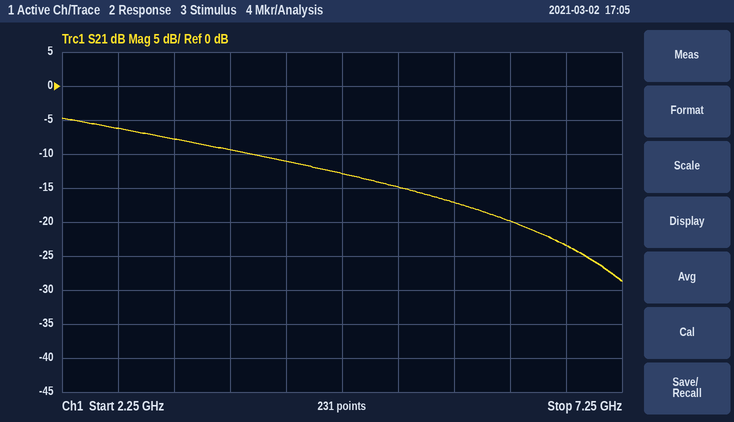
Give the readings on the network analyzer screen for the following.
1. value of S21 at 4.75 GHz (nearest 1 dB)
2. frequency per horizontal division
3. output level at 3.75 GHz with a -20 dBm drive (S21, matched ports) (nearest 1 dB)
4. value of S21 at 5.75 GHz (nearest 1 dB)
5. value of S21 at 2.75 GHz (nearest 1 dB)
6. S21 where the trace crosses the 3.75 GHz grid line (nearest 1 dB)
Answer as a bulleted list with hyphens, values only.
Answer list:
- -13 dB
- 500 MHz
- -29 dBm
- -17 dB
- -6 dB
- -9 dB
